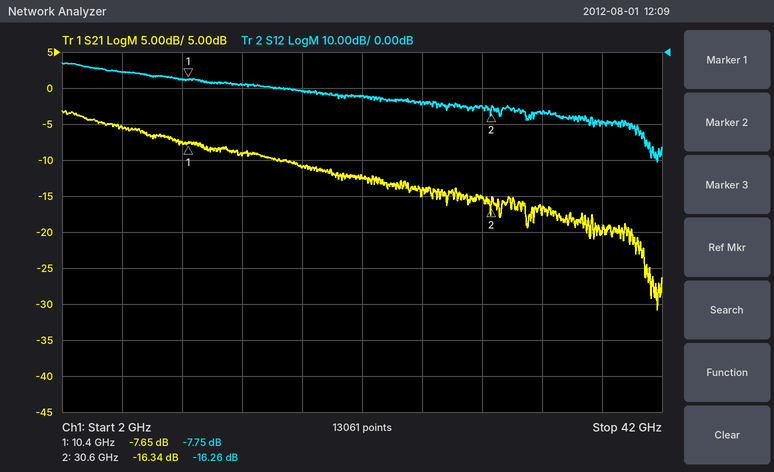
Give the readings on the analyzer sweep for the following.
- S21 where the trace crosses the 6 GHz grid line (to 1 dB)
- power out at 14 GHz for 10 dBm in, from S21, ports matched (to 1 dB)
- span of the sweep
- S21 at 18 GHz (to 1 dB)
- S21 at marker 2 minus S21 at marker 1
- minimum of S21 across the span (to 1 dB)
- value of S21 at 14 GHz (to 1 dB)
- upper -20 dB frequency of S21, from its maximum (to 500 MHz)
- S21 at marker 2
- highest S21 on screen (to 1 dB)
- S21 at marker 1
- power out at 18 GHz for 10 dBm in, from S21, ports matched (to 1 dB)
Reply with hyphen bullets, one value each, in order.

- -5 dB
- 1 dBm
- 40 GHz
- -11 dB
- -8.69 dB
- -31 dB
- -9 dB
- 40.5 GHz
- -16.34 dB
- -3 dB
- -7.65 dB
- -1 dBm
